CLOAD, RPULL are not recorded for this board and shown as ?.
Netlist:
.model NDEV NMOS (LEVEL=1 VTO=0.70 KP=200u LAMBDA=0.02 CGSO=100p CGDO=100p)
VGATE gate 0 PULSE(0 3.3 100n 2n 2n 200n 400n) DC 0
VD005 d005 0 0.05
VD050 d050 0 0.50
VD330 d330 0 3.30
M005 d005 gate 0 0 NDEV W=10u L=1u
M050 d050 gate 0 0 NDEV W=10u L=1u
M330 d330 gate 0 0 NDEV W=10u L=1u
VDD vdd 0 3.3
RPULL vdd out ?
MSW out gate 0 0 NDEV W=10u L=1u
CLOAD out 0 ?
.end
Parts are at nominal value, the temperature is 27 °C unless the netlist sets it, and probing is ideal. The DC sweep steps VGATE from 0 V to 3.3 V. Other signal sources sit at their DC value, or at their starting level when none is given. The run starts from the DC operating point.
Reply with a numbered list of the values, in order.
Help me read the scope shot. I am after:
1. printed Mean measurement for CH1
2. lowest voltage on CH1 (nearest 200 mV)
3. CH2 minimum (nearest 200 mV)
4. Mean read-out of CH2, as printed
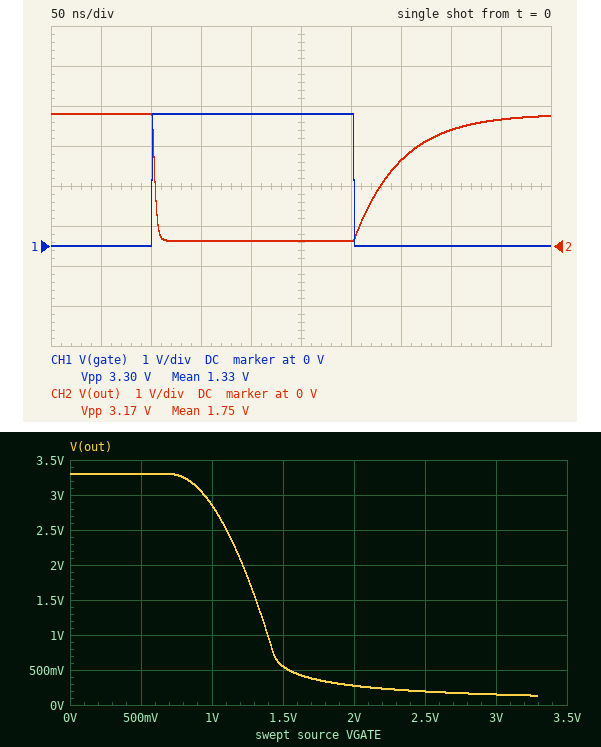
1. 1.33 V
2. 0 V
3. 200 mV
4. 1.75 V
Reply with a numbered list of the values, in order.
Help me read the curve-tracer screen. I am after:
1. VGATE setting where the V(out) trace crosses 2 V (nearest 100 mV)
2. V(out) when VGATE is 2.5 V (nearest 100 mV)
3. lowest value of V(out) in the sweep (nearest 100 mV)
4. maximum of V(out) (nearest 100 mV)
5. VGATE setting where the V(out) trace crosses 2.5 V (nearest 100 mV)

1. 1.2 V
2. 200 mV
3. 100 mV
4. 3.3 V
5. 1.1 V
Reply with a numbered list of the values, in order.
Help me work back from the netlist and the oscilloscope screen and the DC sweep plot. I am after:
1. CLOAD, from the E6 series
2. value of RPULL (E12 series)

1. 10 pF
2. 4.7 kΩ
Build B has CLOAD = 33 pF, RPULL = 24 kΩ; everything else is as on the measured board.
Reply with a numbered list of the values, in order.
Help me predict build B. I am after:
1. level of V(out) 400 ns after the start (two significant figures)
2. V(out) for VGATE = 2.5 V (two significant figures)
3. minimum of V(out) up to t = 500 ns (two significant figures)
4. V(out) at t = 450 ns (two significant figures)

1. 400 mV
2. 38 mV
3. 26 mV
4. 580 mV
